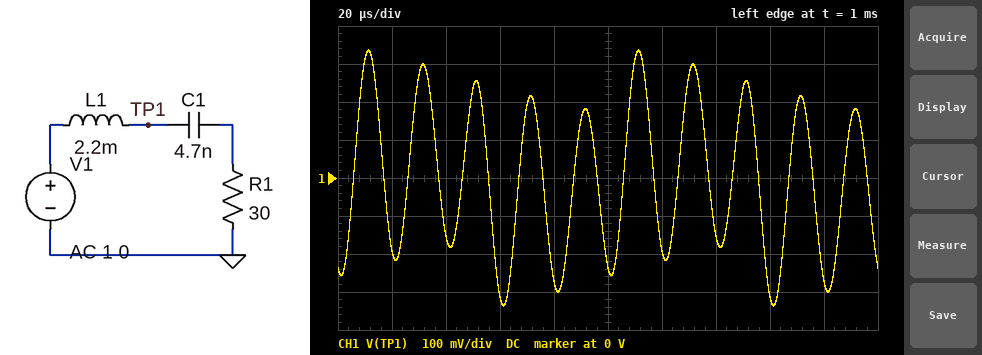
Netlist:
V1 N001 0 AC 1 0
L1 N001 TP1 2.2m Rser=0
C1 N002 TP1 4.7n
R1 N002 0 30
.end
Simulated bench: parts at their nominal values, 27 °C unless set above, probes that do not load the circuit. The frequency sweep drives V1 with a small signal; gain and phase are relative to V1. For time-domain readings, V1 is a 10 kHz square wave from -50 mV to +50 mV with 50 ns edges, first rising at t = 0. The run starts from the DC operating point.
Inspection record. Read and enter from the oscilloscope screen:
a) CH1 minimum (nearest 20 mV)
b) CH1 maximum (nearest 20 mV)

-340 mV
340 mV
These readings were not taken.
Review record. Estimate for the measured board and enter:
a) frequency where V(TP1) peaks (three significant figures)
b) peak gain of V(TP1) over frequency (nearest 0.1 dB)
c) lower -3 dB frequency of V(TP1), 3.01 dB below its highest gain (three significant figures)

49.5 kHz
27.2 dB
48.4 kHz
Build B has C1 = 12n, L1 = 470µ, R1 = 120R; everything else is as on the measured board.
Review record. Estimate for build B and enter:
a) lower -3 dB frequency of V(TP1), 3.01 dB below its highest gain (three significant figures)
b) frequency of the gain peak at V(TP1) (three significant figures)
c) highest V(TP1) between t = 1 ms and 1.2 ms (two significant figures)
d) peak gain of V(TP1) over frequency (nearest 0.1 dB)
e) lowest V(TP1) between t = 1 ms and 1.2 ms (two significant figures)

38.4 kHz
62.3 kHz
95 mV
5.9 dB
-95 mV
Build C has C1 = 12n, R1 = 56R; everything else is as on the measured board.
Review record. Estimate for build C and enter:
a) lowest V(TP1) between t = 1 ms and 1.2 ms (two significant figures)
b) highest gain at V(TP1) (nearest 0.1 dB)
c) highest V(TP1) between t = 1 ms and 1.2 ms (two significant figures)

-210 mV
17.8 dB
210 mV
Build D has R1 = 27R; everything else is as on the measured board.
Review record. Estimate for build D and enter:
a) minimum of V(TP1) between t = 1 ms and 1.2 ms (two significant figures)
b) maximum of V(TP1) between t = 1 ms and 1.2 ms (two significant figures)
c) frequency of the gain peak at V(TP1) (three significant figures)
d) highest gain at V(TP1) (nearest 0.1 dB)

-360 mV
360 mV
49.5 kHz
28.1 dB
